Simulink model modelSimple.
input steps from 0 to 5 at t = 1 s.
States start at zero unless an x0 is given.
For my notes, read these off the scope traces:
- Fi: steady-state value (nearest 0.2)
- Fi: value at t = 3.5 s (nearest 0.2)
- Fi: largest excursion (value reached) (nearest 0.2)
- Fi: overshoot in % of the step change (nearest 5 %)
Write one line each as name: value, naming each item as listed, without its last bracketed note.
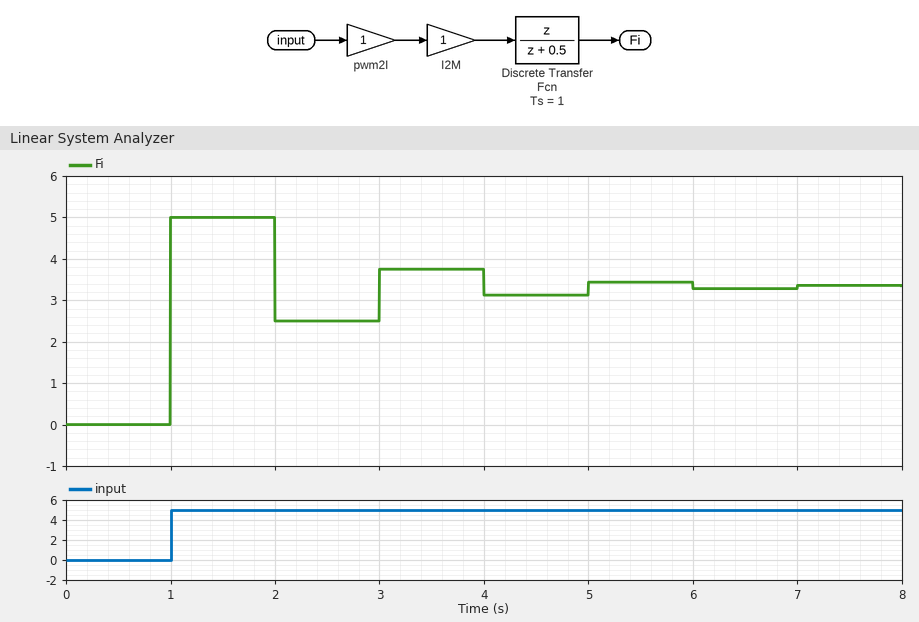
Fi: steady-state value: 3.4
Fi: value at t = 3.5 s: 3.8
Fi: largest excursion (value reached): 5.0
Fi: overshoot in % of the step change: 50 %
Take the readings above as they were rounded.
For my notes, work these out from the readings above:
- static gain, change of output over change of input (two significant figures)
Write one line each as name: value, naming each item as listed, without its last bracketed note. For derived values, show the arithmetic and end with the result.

static gain, change of output over change of input: (3.4 - 0) / (5 - 0) = 0.68
